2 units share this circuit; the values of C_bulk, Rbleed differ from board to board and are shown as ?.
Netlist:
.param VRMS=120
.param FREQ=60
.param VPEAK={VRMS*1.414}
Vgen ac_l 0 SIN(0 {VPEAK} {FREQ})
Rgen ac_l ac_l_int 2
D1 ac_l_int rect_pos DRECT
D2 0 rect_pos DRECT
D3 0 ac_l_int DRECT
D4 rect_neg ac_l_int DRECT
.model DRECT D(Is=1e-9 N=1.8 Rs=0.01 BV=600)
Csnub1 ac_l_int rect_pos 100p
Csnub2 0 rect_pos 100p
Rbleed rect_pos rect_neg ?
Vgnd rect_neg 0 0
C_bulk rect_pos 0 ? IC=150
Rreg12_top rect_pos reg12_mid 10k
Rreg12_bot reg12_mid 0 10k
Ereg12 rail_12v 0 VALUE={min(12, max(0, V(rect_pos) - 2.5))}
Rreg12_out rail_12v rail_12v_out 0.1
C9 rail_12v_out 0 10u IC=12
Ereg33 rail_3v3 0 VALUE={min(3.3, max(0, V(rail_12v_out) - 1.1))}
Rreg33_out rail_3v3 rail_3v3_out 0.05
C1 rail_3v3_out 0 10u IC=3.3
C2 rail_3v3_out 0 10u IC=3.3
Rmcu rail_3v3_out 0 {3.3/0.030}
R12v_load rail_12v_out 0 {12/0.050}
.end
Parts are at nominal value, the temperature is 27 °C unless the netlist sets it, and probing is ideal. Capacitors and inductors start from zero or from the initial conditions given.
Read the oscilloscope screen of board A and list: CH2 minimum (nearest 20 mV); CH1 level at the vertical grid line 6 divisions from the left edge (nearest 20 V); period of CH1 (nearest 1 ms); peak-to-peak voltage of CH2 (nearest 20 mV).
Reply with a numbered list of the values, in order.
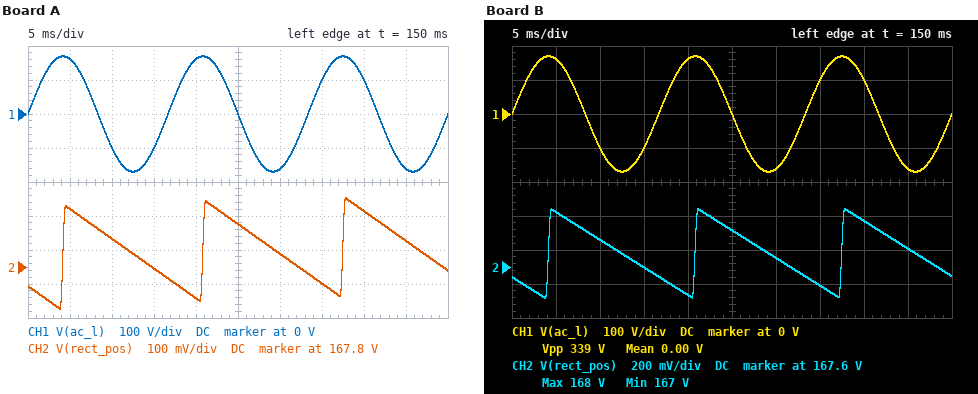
1. 167.68 V
2. -160 V
3. 17 ms
4. 320 mV
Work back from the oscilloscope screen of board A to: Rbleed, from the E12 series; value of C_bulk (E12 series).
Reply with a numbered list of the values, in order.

1. 120 kΩ
2. 560 µF
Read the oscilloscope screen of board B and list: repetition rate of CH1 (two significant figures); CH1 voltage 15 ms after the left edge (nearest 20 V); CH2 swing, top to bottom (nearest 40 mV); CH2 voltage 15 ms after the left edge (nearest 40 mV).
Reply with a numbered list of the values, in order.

1. 60 Hz
2. -100 V
3. 520 mV
4. 167.60 V
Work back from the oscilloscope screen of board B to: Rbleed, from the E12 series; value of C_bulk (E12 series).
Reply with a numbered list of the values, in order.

1. 39 kΩ
2. 390 µF
